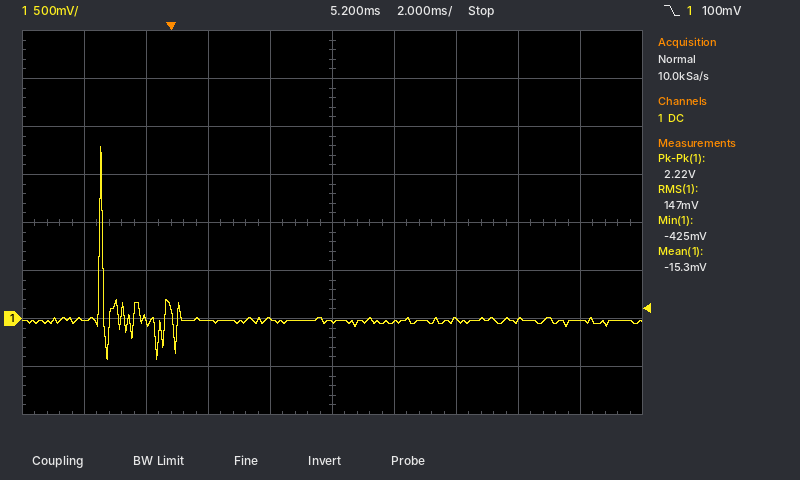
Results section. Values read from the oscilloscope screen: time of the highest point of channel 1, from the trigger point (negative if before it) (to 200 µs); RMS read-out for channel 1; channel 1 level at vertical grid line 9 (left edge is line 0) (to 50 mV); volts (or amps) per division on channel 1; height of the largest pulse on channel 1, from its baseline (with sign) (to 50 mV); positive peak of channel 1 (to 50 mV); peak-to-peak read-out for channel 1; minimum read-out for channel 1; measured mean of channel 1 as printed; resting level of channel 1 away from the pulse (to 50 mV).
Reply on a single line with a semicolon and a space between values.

-2.2 ms; 147 mV; 0 mV; 500 mV; +1.80 V; 1.80 V; 2.22 V; -425 mV; -15.3 mV; 0 mV
